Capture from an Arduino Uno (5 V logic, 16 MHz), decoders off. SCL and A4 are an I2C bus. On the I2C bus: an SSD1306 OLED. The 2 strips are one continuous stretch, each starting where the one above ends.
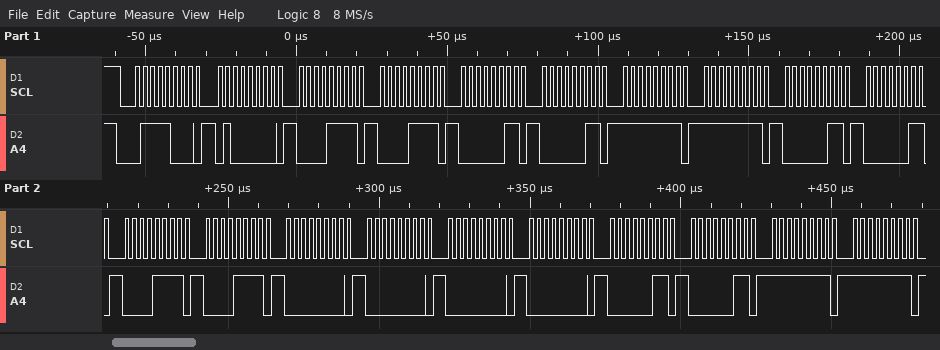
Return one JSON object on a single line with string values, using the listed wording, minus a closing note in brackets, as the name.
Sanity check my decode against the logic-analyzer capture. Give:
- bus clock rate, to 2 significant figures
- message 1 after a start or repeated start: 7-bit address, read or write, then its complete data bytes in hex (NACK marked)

{"bus clock rate, to 2 significant figures": "400 kHz", "message 1 after a start or repeated start: 7-bit address, read or write, then its complete data bytes in hex": "0x3C write: 40 0F 0F 03 03 FF FF 03 03 0F 0F 00 00 00 00 03 03 FF FF"}
